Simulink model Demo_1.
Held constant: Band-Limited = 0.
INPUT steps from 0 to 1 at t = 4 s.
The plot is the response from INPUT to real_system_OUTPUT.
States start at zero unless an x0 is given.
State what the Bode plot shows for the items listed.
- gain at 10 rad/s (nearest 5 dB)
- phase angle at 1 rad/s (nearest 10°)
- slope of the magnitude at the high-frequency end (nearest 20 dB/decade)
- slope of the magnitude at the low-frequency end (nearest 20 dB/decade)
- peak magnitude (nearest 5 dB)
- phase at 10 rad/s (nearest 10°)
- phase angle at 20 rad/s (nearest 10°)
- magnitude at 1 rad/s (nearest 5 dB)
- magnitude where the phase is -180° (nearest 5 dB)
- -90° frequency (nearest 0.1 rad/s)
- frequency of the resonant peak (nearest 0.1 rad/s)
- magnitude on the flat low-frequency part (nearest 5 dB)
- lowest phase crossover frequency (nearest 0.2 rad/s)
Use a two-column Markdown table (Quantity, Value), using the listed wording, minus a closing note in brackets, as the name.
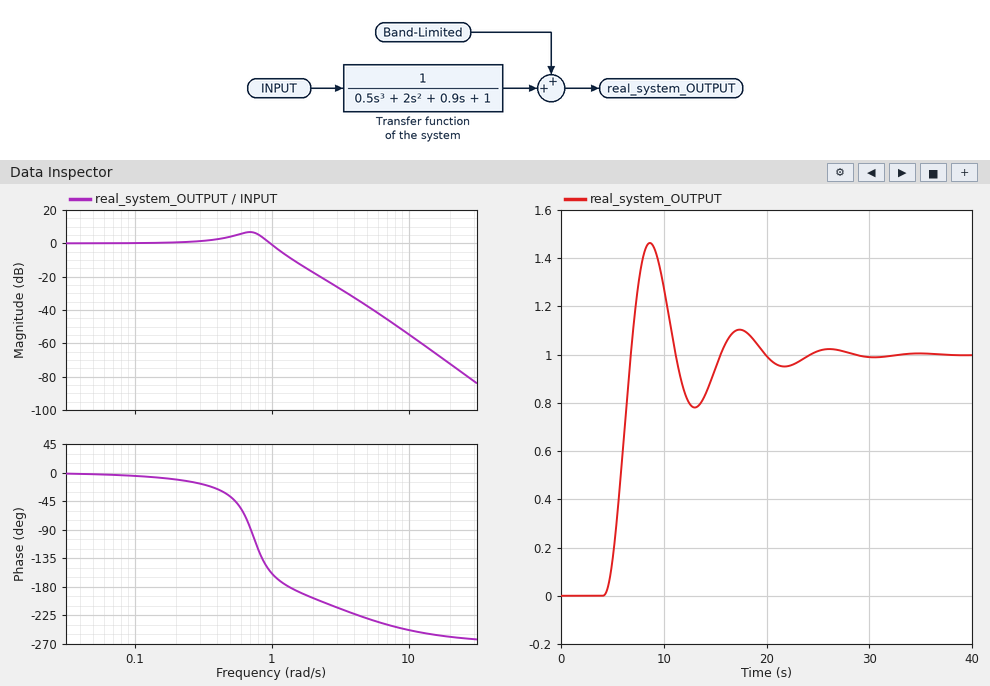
| Quantity | Value |
|---|---|
| gain at 10 rad/s | -55 dB |
| phase angle at 1 rad/s | -160° |
| slope of the magnitude at the high-frequency end | -60 dB/decade |
| slope of the magnitude at the low-frequency end | 0 dB/decade |
| peak magnitude | 5 dB |
| phase at 10 rad/s | -250° |
| phase angle at 20 rad/s | -260° |
| magnitude at 1 rad/s | 0 dB |
| magnitude where the phase is -180° | -10 dB |
| -90° frequency | 0.7 rad/s |
| frequency of the resonant peak | 0.7 rad/s |
| magnitude on the flat low-frequency part | 0 dB |
| lowest phase crossover frequency | 1.4 rad/s |
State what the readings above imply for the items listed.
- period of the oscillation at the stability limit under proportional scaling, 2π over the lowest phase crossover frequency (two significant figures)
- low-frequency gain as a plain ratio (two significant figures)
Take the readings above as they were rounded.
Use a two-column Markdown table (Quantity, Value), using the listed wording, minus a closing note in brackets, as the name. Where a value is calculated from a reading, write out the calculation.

| Quantity | Value |
|---|---|
| period of the oscillation at the stability limit under proportional scaling, 2π over the lowest phase crossover frequency | 2π / 1.4 = 4.5 s |
| low-frequency gain as a plain ratio | 10^(0 / 20) = 1.0 |
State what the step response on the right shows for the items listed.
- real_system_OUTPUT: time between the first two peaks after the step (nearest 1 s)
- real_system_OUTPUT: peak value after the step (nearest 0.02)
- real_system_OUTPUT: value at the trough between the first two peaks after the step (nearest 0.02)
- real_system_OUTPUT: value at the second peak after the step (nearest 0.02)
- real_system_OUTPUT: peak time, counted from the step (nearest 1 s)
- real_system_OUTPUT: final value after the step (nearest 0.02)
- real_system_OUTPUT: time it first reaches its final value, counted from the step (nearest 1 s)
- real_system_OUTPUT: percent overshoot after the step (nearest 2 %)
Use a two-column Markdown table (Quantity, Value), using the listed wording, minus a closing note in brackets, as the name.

| Quantity | Value |
|---|---|
| real_system_OUTPUT: time between the first two peaks after the step | 9 s |
| real_system_OUTPUT: peak value after the step | 1.46 |
| real_system_OUTPUT: value at the trough between the first two peaks after the step | 0.78 |
| real_system_OUTPUT: value at the second peak after the step | 1.10 |
| real_system_OUTPUT: peak time, counted from the step | 5 s |
| real_system_OUTPUT: final value after the step | 1.00 |
| real_system_OUTPUT: time it first reaches its final value, counted from the step | 3 s |
| real_system_OUTPUT: percent overshoot after the step | 46 % |
